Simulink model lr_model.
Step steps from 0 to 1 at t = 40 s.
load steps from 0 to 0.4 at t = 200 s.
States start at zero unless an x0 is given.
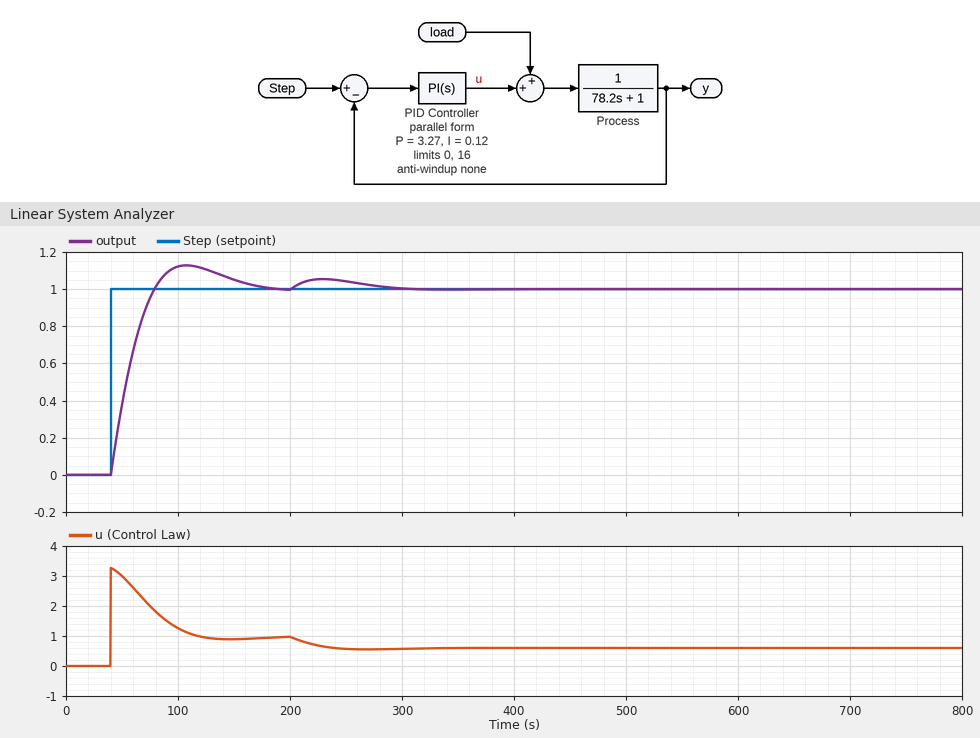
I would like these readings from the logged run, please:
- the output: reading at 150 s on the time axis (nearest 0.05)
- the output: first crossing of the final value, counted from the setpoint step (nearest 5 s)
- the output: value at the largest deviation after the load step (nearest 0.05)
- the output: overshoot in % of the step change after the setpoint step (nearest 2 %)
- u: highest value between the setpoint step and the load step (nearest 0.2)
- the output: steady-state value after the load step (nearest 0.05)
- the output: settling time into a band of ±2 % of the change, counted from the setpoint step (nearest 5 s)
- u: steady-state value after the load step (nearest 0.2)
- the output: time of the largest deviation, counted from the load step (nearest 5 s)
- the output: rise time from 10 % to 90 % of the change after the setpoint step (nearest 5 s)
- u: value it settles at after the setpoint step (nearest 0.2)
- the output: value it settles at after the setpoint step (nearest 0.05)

1.05
40 s
1.05
12 %
3.2
1.00
130 s
0.6
30 s
30 s
1.0
1.00
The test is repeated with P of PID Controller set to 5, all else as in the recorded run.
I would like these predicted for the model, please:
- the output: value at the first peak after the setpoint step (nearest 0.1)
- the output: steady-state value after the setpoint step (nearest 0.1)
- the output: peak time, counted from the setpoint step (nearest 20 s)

1.1
1.0
60 s
